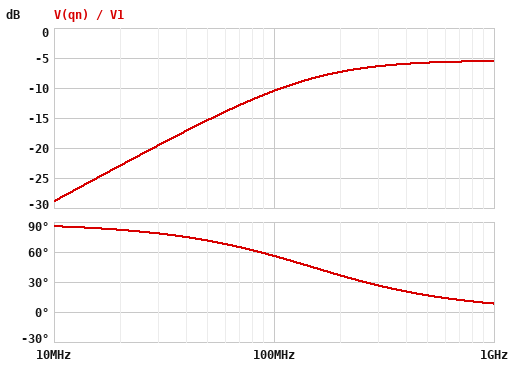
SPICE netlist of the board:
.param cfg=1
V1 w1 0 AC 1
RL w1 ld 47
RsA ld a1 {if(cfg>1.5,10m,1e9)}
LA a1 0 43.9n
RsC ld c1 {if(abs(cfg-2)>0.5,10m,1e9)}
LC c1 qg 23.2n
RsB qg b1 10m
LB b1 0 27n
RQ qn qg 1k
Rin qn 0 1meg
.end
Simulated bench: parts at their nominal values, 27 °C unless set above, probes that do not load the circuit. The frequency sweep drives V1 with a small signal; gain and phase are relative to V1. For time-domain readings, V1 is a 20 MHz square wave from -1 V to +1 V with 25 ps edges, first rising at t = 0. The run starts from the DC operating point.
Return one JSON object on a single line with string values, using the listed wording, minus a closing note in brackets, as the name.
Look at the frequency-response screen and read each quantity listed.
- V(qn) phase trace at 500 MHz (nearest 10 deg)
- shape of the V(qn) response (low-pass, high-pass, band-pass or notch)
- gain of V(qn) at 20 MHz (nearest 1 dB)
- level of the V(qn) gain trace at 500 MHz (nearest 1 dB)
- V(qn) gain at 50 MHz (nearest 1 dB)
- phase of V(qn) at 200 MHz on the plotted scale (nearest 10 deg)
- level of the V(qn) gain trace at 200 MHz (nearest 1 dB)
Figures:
{"V(qn) phase trace at 500 MHz": "20 deg", "shape of the V(qn) response": "high-pass", "gain of V(qn) at 20 MHz": "-23 dB", "level of the V(qn) gain trace at 500 MHz": "-6 dB", "V(qn) gain at 50 MHz": "-15 dB", "phase of V(qn) at 200 MHz on the plotted scale": "40 deg", "level of the V(qn) gain trace at 200 MHz": "-7 dB"}
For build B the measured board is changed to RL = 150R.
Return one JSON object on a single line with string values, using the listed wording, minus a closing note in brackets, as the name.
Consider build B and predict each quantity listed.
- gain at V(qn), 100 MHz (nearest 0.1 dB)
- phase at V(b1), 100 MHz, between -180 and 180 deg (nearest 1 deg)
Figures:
{"gain at V(qn), 100 MHz": "-19.1 dB", "phase at V(b1), 100 MHz, between -180 and 180 deg": "78 deg"}
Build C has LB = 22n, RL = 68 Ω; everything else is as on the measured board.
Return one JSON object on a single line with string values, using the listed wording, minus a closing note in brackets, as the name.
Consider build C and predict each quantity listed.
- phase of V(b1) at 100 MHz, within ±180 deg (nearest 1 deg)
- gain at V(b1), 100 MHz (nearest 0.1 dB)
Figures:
{"phase of V(b1) at 100 MHz, within ±180 deg": "67 deg", "gain at V(b1), 100 MHz": "-14.5 dB"}
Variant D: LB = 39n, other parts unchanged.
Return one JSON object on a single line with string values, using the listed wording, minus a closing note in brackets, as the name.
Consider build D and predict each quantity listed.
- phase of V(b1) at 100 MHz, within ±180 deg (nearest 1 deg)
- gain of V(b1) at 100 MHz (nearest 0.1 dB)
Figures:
{"phase of V(b1) at 100 MHz, within ±180 deg": "50 deg", "gain of V(b1) at 100 MHz": "-7.9 dB"}
